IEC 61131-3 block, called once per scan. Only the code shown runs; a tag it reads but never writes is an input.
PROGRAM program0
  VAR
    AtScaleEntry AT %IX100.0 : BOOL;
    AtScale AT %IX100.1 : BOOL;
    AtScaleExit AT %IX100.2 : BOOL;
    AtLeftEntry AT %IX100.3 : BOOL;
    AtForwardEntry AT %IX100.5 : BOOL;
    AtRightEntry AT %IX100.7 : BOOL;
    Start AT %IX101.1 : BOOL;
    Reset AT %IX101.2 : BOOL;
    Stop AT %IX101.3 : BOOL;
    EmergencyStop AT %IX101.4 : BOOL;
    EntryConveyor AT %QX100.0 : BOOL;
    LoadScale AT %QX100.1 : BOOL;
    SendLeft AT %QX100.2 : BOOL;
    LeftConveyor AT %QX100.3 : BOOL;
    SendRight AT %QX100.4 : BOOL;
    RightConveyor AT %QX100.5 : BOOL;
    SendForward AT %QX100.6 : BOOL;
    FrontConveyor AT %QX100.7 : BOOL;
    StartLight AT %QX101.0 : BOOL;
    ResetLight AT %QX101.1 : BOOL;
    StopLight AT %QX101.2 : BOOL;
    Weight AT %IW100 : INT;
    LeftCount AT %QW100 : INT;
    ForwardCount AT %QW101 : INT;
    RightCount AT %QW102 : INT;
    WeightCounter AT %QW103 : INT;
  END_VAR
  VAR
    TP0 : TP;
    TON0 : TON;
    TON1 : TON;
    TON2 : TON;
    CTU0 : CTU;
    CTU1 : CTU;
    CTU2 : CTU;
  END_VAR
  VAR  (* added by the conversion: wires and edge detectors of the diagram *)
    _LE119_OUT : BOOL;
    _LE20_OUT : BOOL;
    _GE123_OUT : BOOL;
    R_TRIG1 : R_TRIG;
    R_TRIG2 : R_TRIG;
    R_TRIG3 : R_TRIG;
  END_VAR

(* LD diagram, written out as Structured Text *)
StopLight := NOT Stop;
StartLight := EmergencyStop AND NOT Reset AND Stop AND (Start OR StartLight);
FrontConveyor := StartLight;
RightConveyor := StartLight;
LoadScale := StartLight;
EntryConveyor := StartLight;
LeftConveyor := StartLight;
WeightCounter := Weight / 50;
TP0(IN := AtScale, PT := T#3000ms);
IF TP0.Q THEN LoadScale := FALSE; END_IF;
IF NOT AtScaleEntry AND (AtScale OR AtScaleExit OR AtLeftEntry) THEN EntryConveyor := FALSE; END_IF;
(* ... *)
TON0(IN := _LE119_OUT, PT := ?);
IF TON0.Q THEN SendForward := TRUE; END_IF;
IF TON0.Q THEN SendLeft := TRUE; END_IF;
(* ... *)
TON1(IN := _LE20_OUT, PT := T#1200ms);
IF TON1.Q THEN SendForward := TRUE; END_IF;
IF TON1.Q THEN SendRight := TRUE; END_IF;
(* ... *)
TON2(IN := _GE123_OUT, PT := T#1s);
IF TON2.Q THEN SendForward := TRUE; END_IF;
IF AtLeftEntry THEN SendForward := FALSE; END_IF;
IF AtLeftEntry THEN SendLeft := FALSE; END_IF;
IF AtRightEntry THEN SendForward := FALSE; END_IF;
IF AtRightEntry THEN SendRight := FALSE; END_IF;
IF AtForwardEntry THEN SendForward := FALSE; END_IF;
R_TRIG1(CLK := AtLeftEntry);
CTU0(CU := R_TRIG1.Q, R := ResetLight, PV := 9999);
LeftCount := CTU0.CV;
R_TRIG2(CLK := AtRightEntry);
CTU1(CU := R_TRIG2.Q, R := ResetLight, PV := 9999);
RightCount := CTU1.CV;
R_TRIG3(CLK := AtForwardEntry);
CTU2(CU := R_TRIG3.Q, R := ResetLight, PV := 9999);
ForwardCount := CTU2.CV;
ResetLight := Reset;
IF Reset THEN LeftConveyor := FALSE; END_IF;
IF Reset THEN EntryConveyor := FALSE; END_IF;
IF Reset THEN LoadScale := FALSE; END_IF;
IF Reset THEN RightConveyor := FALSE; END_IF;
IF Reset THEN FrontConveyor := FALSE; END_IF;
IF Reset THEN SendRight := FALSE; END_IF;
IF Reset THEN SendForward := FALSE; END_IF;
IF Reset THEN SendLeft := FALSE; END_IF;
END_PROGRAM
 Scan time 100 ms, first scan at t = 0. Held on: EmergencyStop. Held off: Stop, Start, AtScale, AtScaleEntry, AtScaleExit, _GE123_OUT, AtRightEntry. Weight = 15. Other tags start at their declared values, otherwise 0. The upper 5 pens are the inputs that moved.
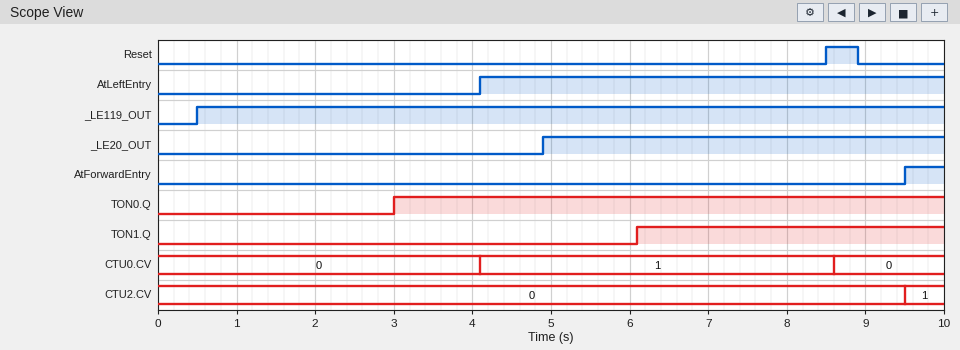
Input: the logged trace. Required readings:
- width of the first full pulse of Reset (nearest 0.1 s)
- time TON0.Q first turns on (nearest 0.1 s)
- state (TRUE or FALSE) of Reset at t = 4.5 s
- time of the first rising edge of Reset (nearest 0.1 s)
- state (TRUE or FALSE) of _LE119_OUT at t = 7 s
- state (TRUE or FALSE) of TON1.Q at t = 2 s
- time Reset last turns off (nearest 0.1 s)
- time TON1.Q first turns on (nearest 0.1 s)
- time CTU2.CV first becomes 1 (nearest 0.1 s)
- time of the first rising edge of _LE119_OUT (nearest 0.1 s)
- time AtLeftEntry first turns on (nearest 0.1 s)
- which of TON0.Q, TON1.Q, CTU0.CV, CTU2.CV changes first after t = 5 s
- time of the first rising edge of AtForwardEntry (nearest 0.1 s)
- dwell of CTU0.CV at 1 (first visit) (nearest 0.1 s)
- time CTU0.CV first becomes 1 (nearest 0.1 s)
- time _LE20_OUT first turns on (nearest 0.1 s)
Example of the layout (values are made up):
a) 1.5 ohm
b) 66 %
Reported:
a) 0.4 s
b) 3.0 s
c) FALSE
d) 8.5 s
e) TRUE
f) FALSE
g) 8.9 s
h) 6.1 s
i) 9.5 s
j) 0.5 s
k) 4.1 s
l) TON1.Q
m) 9.5 s
n) 4.5 s
o) 4.1 s
p) 4.9 s
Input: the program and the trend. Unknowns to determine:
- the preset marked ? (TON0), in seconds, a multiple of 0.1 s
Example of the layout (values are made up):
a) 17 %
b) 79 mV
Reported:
a) 2.5 s
